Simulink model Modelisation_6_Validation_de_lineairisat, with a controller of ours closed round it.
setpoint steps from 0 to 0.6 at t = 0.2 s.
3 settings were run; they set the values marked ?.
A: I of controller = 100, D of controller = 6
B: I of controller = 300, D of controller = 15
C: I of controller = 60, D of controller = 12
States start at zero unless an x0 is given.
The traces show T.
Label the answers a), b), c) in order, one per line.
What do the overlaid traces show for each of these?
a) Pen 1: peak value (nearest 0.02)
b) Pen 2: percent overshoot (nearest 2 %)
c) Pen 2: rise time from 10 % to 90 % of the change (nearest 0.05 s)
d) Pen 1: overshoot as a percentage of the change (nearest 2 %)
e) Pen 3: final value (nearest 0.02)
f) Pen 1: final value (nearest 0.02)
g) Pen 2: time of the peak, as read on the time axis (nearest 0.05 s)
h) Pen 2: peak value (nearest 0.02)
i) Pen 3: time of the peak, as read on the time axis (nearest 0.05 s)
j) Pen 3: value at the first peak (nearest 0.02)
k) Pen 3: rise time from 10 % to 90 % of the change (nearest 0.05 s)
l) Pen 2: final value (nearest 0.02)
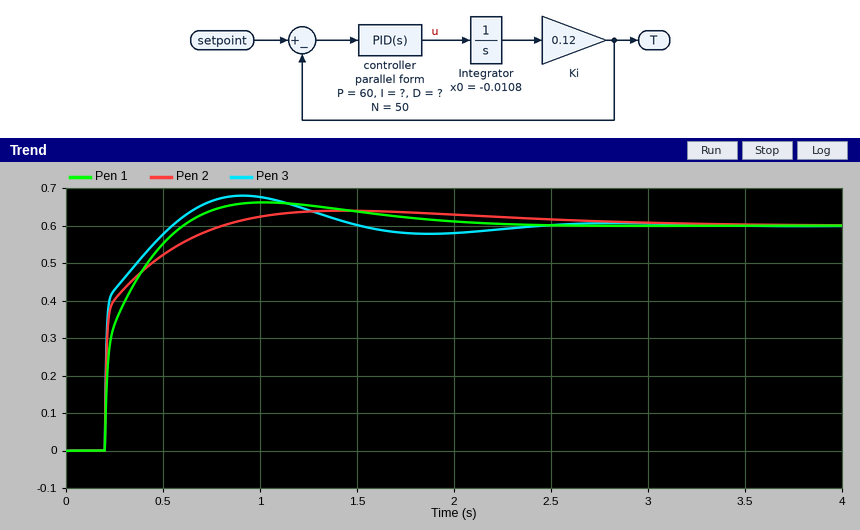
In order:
a) 0.66
b) 6 %
c) 0.35 s
d) 10 %
e) 0.60
f) 0.60
g) 1.45 s
h) 0.64
i) 0.90 s
j) 0.68
k) 0.25 s
l) 0.60
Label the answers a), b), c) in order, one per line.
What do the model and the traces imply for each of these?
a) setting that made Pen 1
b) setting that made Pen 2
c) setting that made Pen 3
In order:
a) A
b) C
c) B
